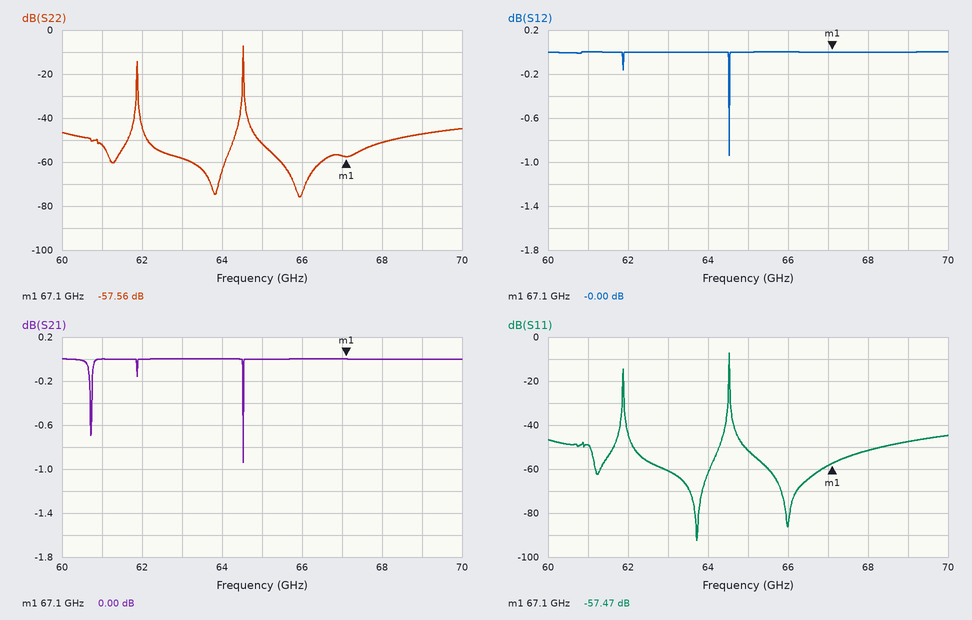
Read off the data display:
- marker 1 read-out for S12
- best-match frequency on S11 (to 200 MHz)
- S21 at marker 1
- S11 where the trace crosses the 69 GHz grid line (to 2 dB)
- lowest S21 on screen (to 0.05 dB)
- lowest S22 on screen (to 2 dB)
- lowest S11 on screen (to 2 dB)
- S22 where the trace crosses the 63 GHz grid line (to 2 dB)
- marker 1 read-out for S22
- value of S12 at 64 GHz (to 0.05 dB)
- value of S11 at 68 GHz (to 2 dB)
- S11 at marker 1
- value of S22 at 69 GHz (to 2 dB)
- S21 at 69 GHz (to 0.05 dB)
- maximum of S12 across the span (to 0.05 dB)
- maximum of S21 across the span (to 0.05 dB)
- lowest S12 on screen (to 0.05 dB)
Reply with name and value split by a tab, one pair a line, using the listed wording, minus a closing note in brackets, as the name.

marker 1 read-out for S12	-0.00 dB
best-match frequency on S11	63.8 GHz
S21 at marker 1	0.00 dB
S11 where the trace crosses the 69 GHz grid line	-48 dB
lowest S21 on screen	-0.95 dB
lowest S22 on screen	-76 dB
lowest S11 on screen	-92 dB
S22 where the trace crosses the 63 GHz grid line	-58 dB
marker 1 read-out for S22	-57.56 dB
value of S12 at 64 GHz	0.00 dB
value of S11 at 68 GHz	-52 dB
S11 at marker 1	-57.47 dB
value of S22 at 69 GHz	-48 dB
S21 at 69 GHz	0.00 dB
maximum of S12 across the span	0.00 dB
maximum of S21 across the span	0.00 dB
lowest S12 on screen	-0.95 dB
